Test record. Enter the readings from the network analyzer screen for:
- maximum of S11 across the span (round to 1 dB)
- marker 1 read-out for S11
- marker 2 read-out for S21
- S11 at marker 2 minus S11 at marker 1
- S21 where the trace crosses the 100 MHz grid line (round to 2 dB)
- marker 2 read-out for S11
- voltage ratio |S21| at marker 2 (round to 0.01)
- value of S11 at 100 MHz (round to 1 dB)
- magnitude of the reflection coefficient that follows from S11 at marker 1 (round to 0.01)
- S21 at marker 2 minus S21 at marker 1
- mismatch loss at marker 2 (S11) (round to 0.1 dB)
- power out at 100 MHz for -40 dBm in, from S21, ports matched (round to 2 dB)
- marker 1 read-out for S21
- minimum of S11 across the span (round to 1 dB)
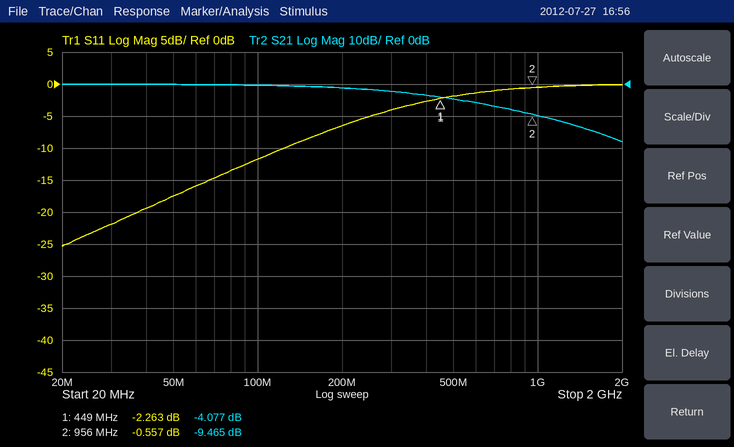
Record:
0 dB
-2.263 dB
-9.465 dB
1.706 dB
0 dB
-0.557 dB
0.34
-12 dB
0.77
-5.388 dB
9.2 dB
-40 dBm
-4.077 dB
-25 dB
